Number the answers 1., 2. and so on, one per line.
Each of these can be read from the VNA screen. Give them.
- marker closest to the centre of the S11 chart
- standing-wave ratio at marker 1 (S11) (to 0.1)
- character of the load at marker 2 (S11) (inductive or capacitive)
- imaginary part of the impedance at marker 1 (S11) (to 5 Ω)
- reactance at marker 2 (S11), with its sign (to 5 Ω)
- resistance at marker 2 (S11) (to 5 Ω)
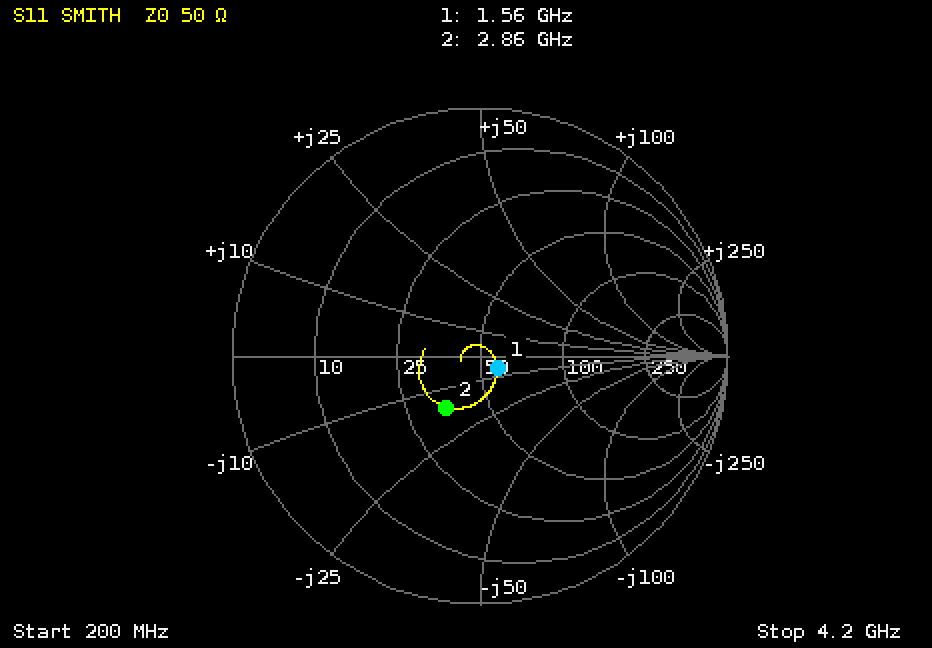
1. marker 1
2. 1.2
3. capacitive
4. -5 Ω
5. -15 Ω
6. 35 Ω
